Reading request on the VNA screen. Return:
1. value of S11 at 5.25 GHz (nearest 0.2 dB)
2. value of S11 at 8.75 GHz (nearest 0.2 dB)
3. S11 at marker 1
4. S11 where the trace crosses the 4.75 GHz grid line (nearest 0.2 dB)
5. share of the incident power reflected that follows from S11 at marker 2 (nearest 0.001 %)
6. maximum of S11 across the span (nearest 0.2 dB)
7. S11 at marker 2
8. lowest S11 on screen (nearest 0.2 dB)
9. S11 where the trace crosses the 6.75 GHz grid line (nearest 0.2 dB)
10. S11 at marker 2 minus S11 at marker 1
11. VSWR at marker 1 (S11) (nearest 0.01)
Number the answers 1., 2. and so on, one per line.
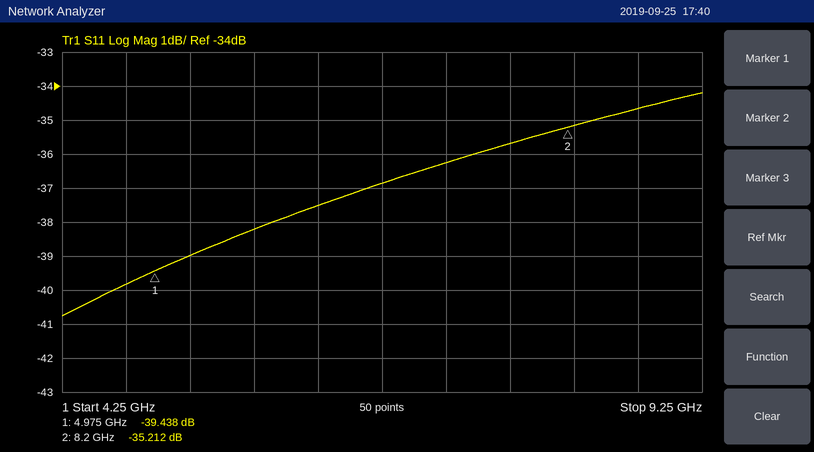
1. -39.0 dB
2. -34.6 dB
3. -39.438 dB
4. -39.8 dB
5. 0.030 %
6. -34.2 dB
7. -35.212 dB
8. -40.8 dB
9. -36.8 dB
10. 4.226 dB
11. 1.02
